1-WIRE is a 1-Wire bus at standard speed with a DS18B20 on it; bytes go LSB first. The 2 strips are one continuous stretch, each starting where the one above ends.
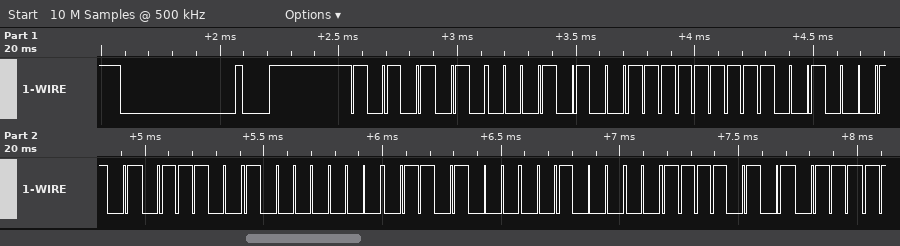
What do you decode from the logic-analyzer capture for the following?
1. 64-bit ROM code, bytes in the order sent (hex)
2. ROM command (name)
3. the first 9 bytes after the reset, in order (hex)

28 FF 89 3A 01 16 04 AF
Match ROM
55 28 FF 89 3A 01 16 04 AF
